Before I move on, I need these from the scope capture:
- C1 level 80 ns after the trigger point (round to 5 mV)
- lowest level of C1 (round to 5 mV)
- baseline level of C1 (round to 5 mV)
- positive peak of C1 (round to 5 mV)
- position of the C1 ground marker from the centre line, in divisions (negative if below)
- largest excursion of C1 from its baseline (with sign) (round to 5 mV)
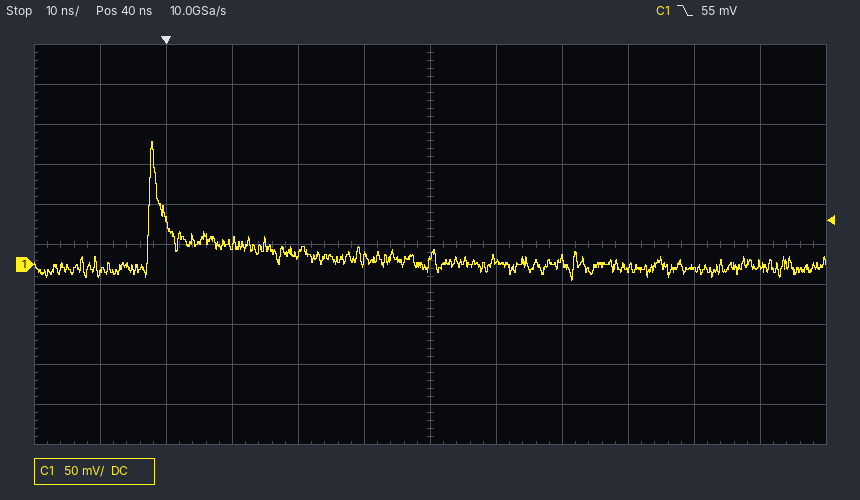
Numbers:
-5 mV
-20 mV
0 mV
155 mV
-0.5 div
+155 mV
